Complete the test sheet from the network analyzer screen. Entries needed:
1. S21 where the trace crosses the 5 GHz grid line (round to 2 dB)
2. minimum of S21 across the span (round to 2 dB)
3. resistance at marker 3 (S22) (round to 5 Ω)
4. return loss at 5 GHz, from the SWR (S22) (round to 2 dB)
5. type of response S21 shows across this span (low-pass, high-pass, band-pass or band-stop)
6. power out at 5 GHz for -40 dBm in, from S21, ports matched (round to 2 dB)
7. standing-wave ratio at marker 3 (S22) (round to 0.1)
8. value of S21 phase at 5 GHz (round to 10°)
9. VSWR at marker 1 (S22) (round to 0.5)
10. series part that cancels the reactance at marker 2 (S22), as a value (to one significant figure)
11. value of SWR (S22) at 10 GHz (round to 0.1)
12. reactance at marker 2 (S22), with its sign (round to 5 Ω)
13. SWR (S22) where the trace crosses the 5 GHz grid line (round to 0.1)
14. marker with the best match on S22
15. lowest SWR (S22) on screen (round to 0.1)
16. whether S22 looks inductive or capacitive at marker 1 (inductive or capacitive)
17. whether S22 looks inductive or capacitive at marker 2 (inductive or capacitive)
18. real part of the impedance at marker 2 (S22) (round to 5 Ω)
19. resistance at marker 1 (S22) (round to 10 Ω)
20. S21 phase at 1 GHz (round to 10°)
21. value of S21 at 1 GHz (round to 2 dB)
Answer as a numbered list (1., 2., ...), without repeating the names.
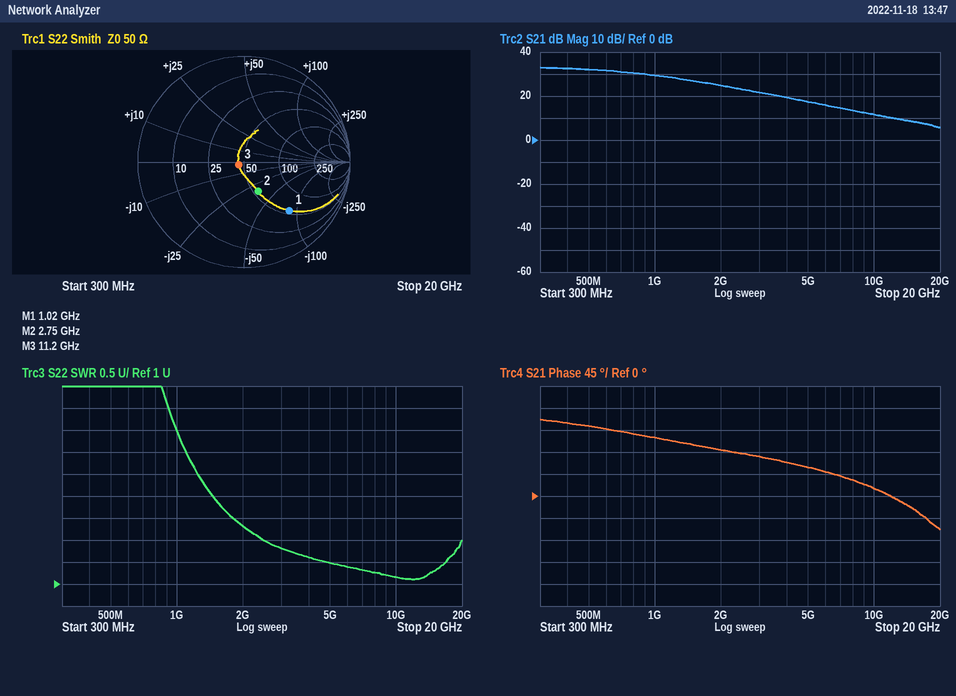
1. 18 dB
2. 6 dB
3. 45 Ω
4. 14 dB
5. low-pass
6. -22 dBm
7. 1.1
8. 60°
9. 4.5
10. 2 nH
11. 1.2
12. -35 Ω
13. 1.5
14. marker 3
15. 1.1
16. capacitive
17. capacitive
18. 55 Ω
19. 60 Ω
20. 120°
21. 30 dB
